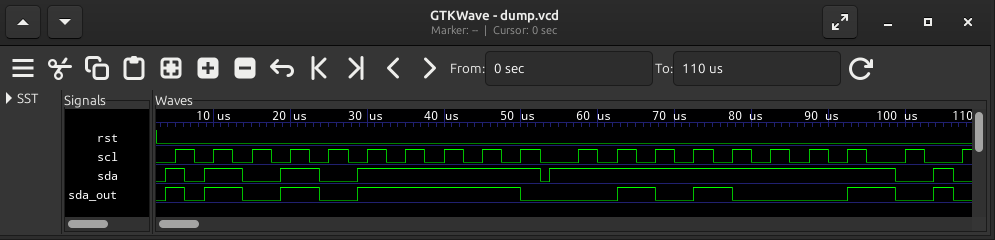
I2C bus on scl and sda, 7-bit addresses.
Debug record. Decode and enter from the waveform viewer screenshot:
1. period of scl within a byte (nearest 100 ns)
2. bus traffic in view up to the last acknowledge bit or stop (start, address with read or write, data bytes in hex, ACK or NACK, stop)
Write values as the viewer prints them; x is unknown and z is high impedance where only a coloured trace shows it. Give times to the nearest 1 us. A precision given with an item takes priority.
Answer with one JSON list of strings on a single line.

["5000 ns", "start, address 57 read NACK, FF ACK"]
